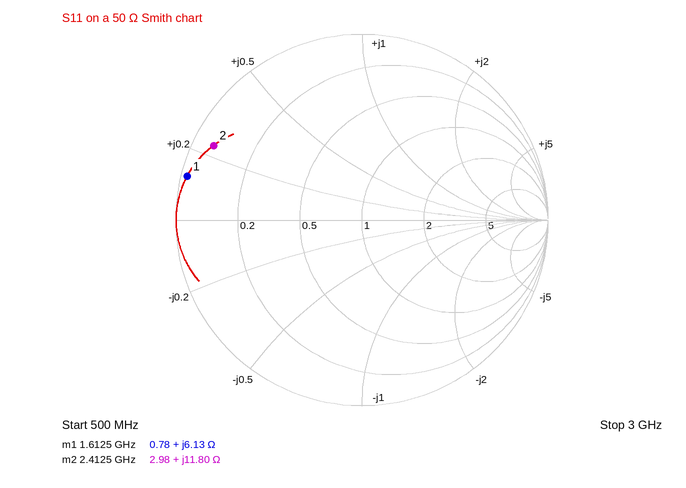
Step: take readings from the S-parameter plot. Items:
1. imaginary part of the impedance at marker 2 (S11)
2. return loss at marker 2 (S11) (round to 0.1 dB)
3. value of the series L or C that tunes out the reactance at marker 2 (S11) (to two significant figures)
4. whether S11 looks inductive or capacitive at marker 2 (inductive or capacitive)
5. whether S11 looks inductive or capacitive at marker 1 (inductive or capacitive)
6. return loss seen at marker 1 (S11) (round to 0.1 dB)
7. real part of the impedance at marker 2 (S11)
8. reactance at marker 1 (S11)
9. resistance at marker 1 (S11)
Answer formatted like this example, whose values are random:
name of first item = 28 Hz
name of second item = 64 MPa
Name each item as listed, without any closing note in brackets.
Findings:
imaginary part of the impedance at marker 2 = +11.80 Ω
return loss at marker 2 (S11) = 1.0 dB
value of the series L or C that tunes out the reactance at marker 2 (S11) = 5.6 pF
whether S11 looks inductive or capacitive at marker 2 = inductive
whether S11 looks inductive or capacitive at marker 1 = inductive
return loss seen at marker 1 (S11) = 0.3 dB
real part of the impedance at marker 2 = 2.98 Ω
reactance at marker 1 = +6.13 Ω
resistance at marker 1 = 0.78 Ω
